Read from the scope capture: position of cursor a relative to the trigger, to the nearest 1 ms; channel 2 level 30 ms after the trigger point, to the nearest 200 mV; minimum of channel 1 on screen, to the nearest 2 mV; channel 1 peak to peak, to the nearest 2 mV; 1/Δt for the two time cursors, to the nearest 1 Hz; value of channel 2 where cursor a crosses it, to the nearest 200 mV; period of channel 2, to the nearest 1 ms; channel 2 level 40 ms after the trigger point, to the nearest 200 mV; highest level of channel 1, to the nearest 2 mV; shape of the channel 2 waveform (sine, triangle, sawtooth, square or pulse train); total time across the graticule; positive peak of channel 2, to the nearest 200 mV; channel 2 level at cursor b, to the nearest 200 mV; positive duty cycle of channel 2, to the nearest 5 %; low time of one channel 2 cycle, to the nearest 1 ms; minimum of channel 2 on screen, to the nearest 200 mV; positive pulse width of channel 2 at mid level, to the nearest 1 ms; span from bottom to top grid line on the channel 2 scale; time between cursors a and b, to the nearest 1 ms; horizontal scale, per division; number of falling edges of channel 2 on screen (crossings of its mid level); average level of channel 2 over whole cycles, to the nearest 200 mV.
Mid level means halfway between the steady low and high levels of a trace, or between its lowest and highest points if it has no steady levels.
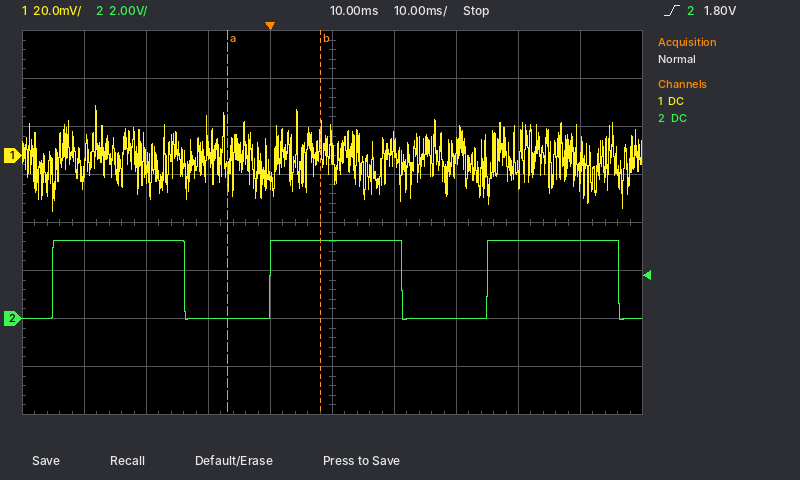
-7 ms
0.0 V
-24 mV
44 mV
67 Hz
0.0 V
35 ms
3.2 V
20 mV
pulse train
100 ms
3.2 V
3.2 V
60 %
14 ms
0.0 V
21 ms
16 V
15 ms
10 ms
3
2.0 V
